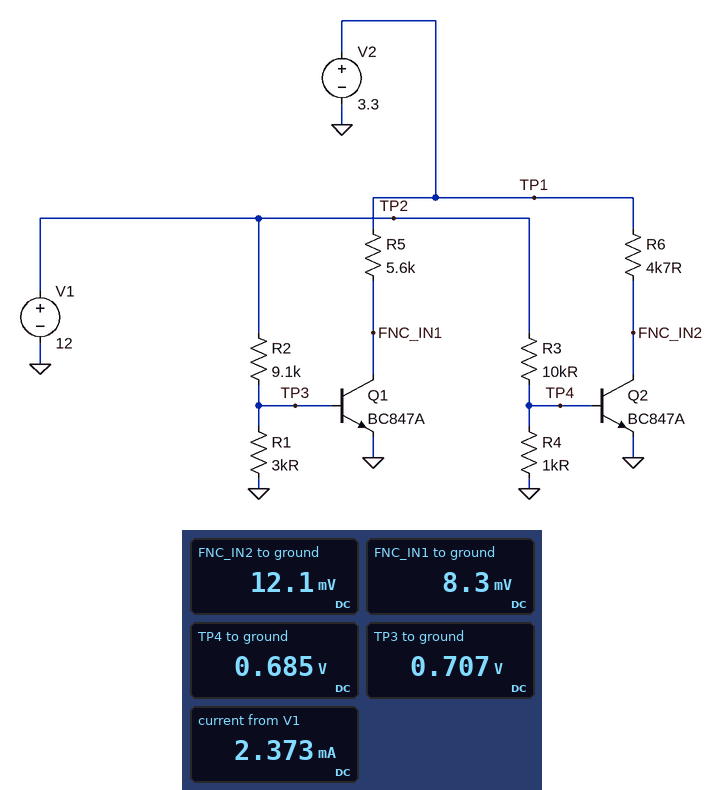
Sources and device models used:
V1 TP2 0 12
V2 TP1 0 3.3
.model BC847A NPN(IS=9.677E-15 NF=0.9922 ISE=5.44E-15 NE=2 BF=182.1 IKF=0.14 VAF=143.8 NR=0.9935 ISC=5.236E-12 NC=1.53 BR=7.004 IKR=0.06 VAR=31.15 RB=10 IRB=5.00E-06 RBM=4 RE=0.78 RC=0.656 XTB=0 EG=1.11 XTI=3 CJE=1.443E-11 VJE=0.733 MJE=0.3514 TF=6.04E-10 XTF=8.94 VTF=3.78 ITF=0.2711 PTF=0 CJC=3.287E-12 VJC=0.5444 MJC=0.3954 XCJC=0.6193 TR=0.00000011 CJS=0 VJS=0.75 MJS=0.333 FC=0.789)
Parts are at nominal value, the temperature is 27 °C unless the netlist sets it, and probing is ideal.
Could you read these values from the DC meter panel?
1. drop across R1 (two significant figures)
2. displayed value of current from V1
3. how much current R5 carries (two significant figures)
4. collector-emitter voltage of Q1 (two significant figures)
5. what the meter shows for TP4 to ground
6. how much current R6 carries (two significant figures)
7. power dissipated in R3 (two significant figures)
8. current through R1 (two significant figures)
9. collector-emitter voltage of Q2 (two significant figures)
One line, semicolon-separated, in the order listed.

710 mV; 2.373 mA; 590 µA; 8.3 mV; 0.685 V; 700 µA; 13 mW; 240 µA; 12 mV
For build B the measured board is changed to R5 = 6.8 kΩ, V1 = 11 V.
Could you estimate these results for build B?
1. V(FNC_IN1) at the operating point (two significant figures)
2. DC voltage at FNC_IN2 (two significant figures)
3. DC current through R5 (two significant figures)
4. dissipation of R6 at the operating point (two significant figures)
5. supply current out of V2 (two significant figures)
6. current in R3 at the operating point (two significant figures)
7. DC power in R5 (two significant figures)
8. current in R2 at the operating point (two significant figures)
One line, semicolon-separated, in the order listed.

7.8 mV; 14 mV; 480 µA; 2.3 mW; 1.2 mA; 1.0 mA; 1.6 mW; 1.1 mA
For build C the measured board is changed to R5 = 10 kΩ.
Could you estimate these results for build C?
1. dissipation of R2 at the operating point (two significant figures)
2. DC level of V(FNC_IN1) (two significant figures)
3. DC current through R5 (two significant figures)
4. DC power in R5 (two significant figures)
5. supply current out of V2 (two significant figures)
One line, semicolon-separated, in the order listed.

14 mW; 6.8 mV; 330 µA; 1.1 mW; 1.0 mA
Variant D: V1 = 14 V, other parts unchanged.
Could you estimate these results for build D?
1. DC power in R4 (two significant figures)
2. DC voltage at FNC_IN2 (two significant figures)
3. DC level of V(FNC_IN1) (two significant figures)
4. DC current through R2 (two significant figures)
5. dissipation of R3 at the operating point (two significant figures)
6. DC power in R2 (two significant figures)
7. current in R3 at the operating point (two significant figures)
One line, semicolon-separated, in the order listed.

480 µW; 10 mV; 8.0 mV; 1.5 mA; 18 mW; 19 mW; 1.3 mA
